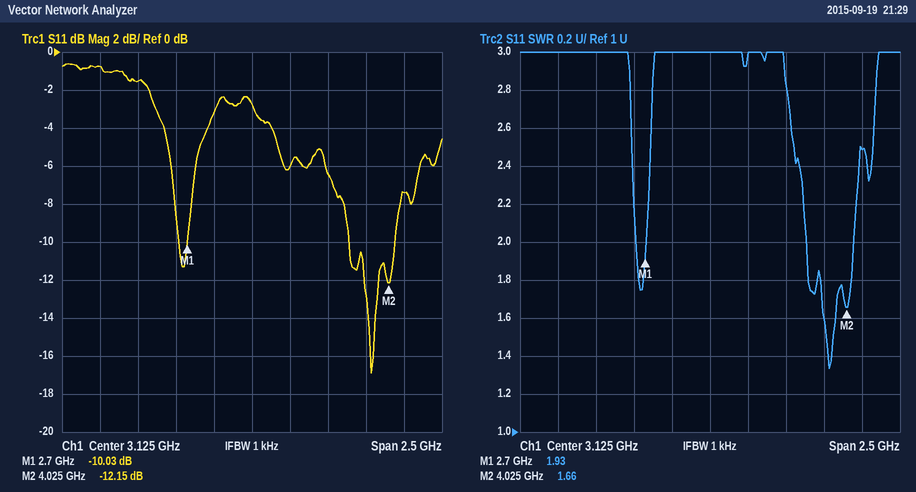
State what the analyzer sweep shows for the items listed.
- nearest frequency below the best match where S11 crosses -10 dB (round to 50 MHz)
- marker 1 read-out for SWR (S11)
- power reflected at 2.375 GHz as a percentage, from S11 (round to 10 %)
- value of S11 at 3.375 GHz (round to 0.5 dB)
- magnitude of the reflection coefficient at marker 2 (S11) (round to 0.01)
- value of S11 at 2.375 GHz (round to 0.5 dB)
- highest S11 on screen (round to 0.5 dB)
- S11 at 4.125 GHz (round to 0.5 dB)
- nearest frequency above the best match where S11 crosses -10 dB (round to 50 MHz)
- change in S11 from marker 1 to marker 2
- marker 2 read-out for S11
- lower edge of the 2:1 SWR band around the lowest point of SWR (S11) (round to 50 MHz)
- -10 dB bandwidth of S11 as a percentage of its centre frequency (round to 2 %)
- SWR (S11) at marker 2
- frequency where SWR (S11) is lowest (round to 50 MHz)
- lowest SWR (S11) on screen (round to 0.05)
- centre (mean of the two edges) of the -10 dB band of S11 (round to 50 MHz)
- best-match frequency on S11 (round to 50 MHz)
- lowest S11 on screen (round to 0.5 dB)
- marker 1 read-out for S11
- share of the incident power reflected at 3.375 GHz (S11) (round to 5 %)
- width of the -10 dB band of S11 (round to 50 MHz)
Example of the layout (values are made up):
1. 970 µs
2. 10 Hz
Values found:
1. 3.75 GHz
2. 1.93
3. 70 %
4. -6.0 dB
5. 0.25
6. -1.5 dB
7. -0.5 dB
8. -7.5 dB
9. 4.05 GHz
10. -2.12 dB
11. -12.15 dB
12. 3.75 GHz
13. 8 %
14. 1.66
15. 3.90 GHz
16. 1.35
17. 3.90 GHz
18. 3.90 GHz
19. -17.0 dB
20. -10.03 dB
21. 25 %
22. 300 MHz
